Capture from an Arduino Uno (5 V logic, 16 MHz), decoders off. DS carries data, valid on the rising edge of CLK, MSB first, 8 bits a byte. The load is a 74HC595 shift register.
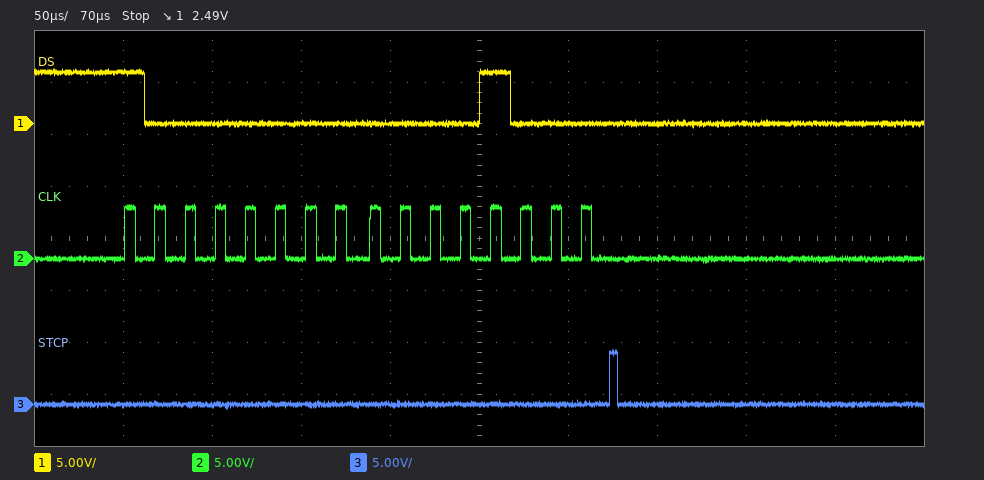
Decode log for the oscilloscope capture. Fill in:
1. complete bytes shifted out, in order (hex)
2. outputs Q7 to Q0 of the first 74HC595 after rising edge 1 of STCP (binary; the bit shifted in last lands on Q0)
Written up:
80 08
00001000
